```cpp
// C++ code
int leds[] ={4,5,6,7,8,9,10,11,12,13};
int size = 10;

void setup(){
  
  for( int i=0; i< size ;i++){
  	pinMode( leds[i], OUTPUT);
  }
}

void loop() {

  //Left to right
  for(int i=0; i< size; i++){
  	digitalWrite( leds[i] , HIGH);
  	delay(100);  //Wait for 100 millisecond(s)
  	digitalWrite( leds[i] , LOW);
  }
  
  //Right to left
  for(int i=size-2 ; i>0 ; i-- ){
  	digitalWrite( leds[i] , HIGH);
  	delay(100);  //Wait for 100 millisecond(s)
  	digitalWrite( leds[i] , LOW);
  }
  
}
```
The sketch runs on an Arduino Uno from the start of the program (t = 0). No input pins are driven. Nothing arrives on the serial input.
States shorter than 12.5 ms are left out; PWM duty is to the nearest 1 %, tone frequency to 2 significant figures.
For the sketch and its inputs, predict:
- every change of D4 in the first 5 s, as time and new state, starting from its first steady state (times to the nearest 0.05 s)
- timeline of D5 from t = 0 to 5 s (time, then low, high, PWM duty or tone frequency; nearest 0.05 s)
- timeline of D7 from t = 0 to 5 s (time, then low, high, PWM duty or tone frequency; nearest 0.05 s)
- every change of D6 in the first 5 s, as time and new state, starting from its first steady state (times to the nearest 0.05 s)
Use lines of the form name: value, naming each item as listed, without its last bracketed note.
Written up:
every change of D4 in the first 5 s, as time and new state, starting from its first steady state: 0 s high; 0.1 s low; 1.8 s high; 1.9 s low; 3.6 s high; 3.7 s low
timeline of D5 from t = 0 to 5 s: 0 s low; 0.1 s high; 0.2 s low; 1.7 s high; 1.8 s low; 1.9 s high; 2 s low; 3.5 s high; 3.6 s low; 3.7 s high; 3.8 s low
timeline of D7 from t = 0 to 5 s: 0 s low; 0.3 s high; 0.4 s low; 1.5 s high; 1.6 s low; 2.1 s high; 2.2 s low; 3.3 s high; 3.4 s low; 3.9 s high; 4 s low
every change of D6 in the first 5 s, as time and new state, starting from its first steady state: 0 s low; 0.2 s high; 0.3 s low; 1.6 s high; 1.7 s low; 2 s high; 2.1 s low; 3.4 s high; 3.5 s low; 3.8 s high; 3.9 s low
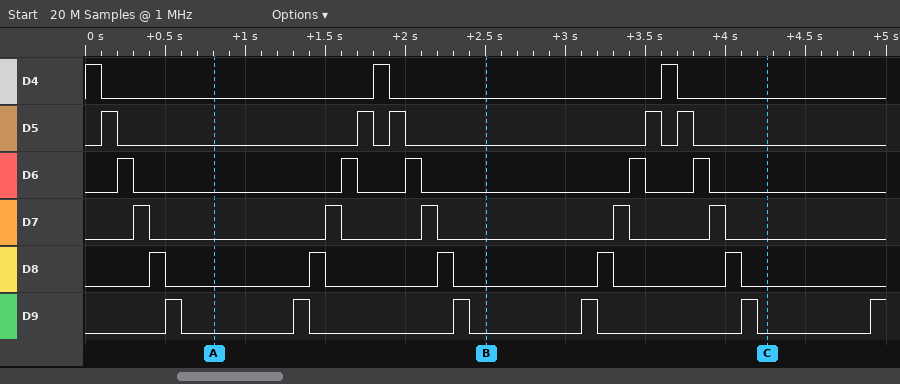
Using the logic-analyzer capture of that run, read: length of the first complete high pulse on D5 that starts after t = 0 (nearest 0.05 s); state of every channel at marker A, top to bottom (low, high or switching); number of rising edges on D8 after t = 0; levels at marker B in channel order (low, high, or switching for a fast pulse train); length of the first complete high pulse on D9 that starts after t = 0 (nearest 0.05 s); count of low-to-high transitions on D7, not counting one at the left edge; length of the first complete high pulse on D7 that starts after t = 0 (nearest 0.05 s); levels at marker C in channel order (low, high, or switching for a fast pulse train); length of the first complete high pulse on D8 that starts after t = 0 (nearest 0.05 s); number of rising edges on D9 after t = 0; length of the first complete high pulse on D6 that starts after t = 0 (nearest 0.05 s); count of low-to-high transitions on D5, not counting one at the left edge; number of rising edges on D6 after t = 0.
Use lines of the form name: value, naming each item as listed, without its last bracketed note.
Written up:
length of the first complete high pulse on D5 that starts after t = 0: 0.10 s
state of every channel at marker A, top to bottom: D4 low, D5 low, D6 low, D7 low, D8 low, D9 low
number of rising edges on D8 after t = 0: 5
levels at marker B in channel order: D4 low, D5 low, D6 low, D7 low, D8 low, D9 low
length of the first complete high pulse on D9 that starts after t = 0: 0.10 s
count of low-to-high transitions on D7, not counting one at the left edge: 5
length of the first complete high pulse on D7 that starts after t = 0: 0.10 s
levels at marker C in channel order: D4 low, D5 low, D6 low, D7 low, D8 low, D9 low
length of the first complete high pulse on D8 that starts after t = 0: 0.10 s
number of rising edges on D9 after t = 0: 6
length of the first complete high pulse on D6 that starts after t = 0: 0.10 s
count of low-to-high transitions on D5, not counting one at the left edge: 5
number of rising edges on D6 after t = 0: 5
